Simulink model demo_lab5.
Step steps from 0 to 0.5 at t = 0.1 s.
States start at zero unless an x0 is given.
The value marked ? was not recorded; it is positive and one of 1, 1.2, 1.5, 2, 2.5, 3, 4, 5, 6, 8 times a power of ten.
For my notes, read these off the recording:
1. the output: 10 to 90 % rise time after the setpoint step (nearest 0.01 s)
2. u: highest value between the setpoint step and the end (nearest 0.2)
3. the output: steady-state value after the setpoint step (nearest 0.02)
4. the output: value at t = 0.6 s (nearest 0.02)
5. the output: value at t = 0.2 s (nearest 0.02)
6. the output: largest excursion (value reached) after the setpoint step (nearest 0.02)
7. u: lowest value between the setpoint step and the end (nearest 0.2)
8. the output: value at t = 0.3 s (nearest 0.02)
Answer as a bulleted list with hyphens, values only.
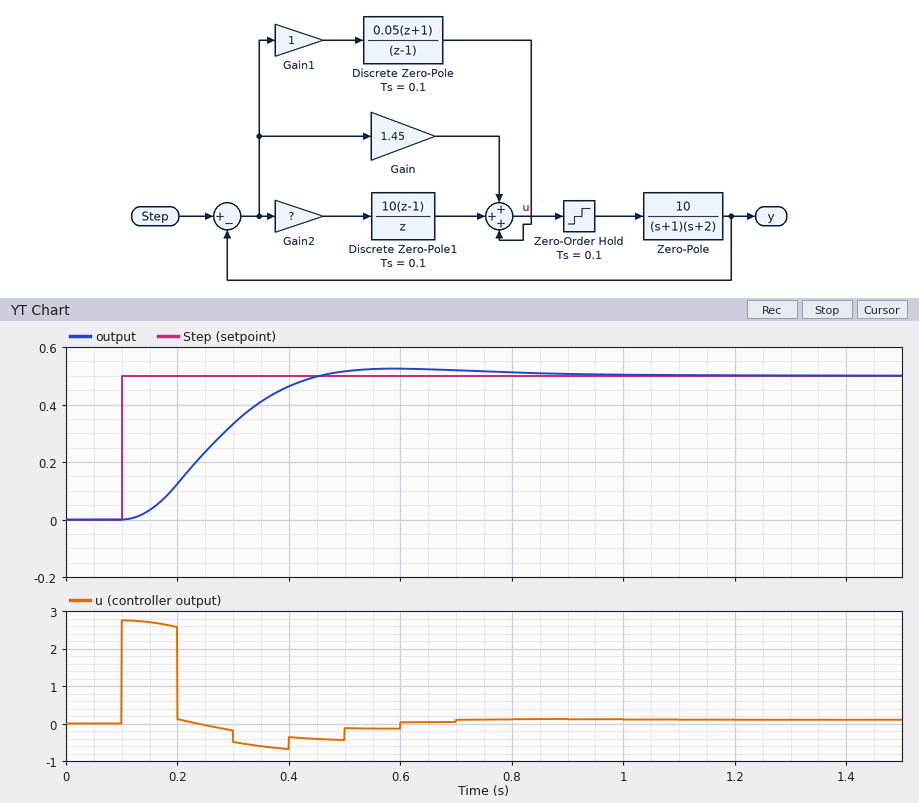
- 0.22 s
- 2.8
- 0.50
- 0.52
- 0.12
- 0.52
- -0.6
- 0.34
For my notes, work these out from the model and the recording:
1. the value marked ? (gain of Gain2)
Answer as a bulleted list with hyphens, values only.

- 0.4
